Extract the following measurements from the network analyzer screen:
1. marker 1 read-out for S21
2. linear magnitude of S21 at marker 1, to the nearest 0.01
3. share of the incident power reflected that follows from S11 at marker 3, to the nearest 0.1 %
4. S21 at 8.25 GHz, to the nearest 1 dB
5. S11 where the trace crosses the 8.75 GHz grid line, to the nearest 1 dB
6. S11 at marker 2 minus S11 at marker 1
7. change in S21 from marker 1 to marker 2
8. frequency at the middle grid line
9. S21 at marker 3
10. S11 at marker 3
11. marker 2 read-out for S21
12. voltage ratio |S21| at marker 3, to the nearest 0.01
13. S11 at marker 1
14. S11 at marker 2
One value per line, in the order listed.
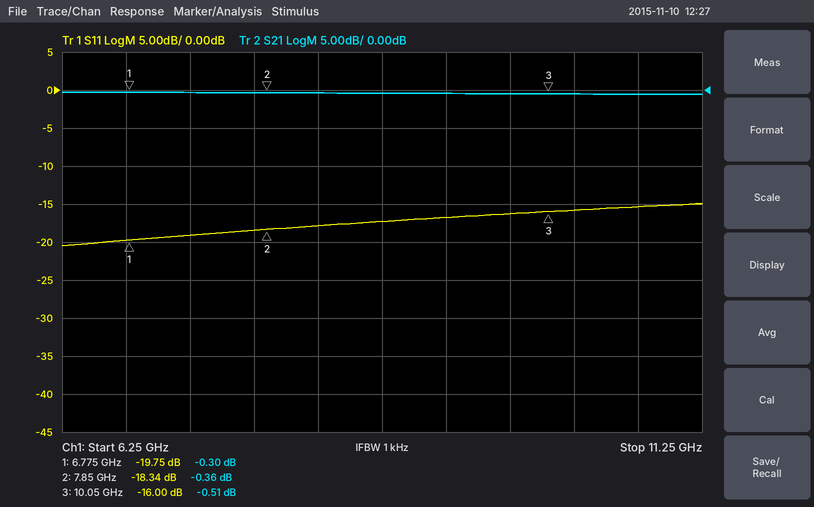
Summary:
-0.30 dB
0.97
2.5 %
0 dB
-17 dB
1.41 dB
-0.06 dB
8.75 GHz
-0.51 dB
-16.00 dB
-0.36 dB
0.94
-19.75 dB
-18.34 dB
